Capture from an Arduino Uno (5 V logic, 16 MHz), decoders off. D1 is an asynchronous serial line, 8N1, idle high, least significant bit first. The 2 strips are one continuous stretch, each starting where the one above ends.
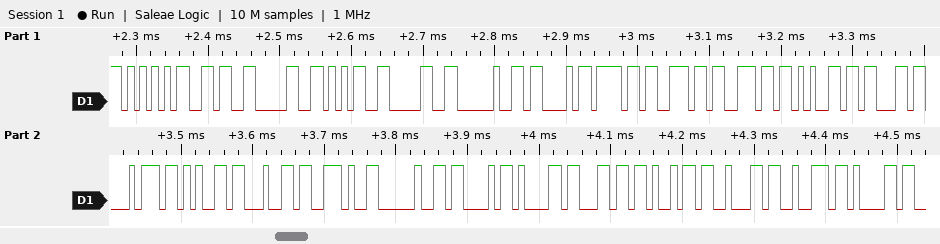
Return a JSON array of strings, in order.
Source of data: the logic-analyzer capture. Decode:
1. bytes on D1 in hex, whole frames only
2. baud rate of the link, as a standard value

["55 36 30 35 30 20 43 6F 6E 6E 65 63 74 65 64 2E 20 43 61 6C 69 62 72 61", "115200 baud"]
